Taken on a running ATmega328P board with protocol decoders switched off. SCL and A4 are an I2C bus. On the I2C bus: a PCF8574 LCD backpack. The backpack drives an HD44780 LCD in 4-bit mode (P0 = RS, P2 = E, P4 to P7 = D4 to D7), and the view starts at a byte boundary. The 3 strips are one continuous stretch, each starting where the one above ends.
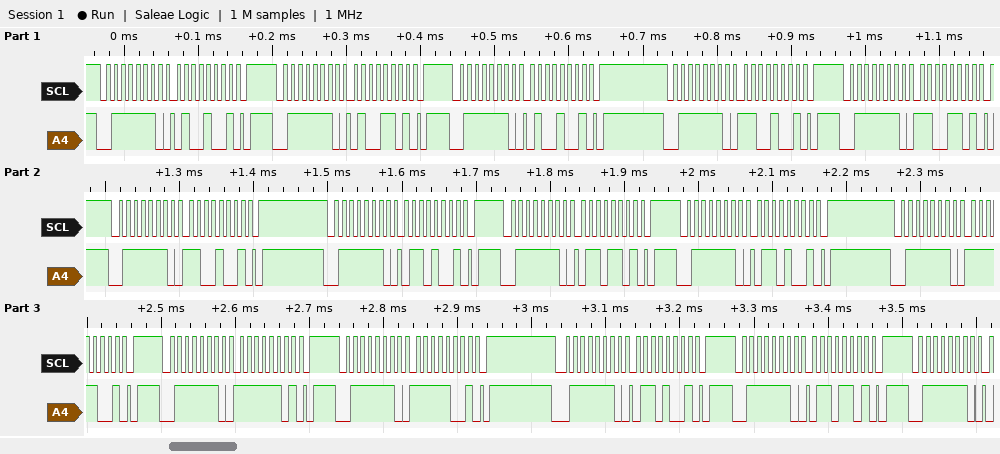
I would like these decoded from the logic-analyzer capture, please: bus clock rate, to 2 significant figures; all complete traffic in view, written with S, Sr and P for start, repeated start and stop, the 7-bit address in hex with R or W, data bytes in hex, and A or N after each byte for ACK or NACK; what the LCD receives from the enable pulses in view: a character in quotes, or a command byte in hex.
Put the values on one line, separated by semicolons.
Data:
100 kHz; S 3FW A 49 A P S 3FW A 4D A P S 3FW A 49 A P S 3FW A C9 A P S 3FW A CD A P S 3FW A C9 A P S 3FW A 69 A P S 3FW A 6D A P S 3FW A 69 A P S 3FW A F9 A P S 3FW A FD A P S 3FW A F9 A P S 3FW A 69 A P S 3FW A 6D A P S 3FW A; 'L' 'o'
